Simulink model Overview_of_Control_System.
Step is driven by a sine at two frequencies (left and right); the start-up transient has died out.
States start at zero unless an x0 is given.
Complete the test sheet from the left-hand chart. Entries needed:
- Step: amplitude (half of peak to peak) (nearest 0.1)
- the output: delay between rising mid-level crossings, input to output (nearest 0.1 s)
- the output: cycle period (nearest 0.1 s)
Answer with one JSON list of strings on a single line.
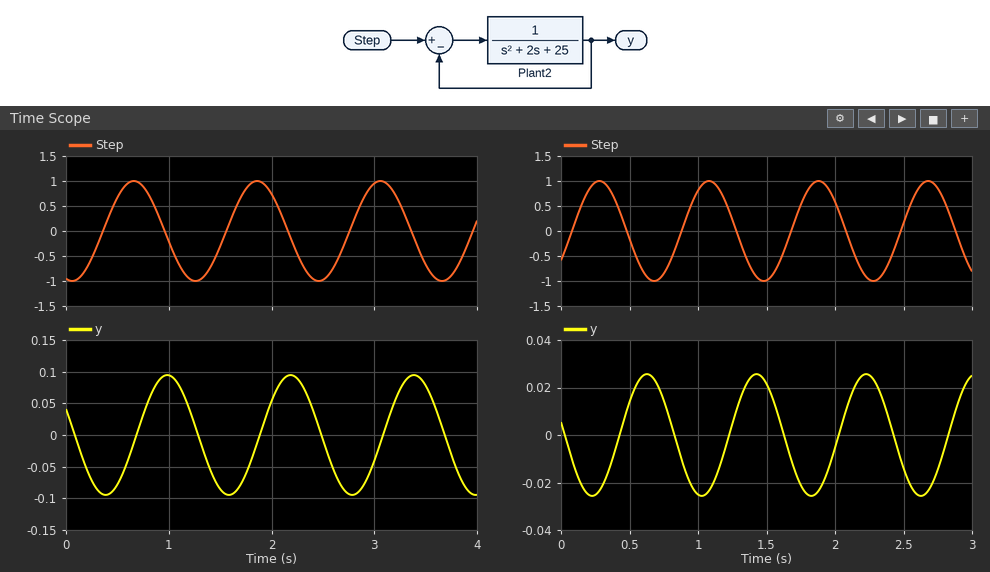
["1.0", "0.3 s", "1.2 s"]
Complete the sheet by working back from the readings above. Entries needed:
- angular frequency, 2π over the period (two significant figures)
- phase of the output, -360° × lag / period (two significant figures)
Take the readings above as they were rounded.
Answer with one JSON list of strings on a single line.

["5.2 rad/s", "-90°"]
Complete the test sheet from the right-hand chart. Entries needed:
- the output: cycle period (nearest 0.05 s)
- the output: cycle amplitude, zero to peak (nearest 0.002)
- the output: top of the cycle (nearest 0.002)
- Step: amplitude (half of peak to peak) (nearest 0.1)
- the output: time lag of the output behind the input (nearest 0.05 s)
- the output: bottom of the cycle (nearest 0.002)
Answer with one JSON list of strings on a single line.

["0.80 s", "0.026", "0.026", "1.0", "0.35 s", "-0.026"]
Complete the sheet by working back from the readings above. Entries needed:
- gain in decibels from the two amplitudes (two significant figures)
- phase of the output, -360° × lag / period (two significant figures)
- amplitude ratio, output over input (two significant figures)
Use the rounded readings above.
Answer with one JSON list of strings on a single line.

["-32 dB", "-160°", "0.026"]
